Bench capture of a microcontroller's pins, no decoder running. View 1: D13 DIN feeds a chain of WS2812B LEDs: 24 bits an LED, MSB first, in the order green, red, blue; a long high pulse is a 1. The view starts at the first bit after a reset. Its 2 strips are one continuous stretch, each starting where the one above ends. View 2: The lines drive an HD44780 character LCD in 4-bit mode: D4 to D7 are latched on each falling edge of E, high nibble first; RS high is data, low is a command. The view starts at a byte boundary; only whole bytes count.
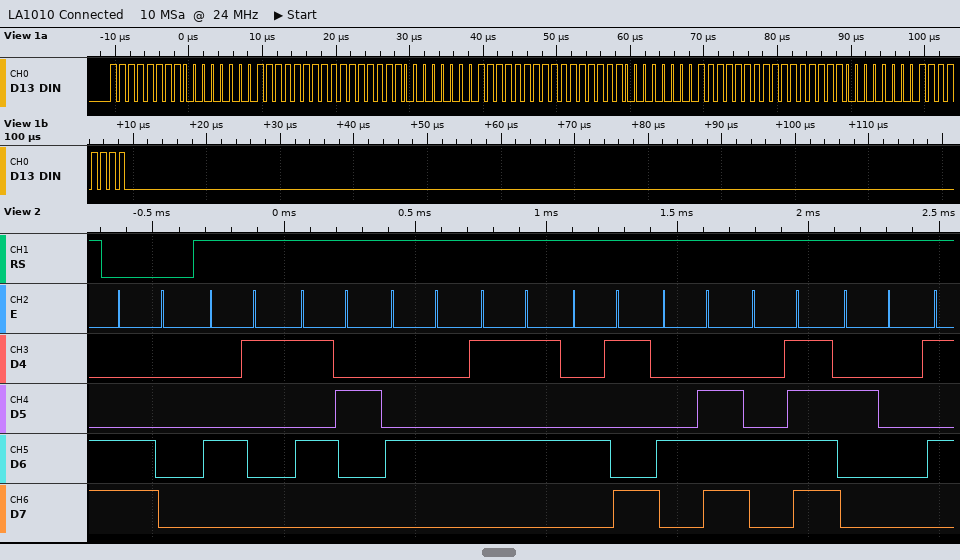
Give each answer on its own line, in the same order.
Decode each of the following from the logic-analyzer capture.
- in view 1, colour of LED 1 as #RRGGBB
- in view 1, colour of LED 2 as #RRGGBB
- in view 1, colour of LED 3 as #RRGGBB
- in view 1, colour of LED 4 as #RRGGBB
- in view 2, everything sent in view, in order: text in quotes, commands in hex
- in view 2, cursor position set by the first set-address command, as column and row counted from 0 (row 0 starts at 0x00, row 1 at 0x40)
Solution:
#00FFFF
#00FFFF
#00FFFF
#00FFFF
0xC0 "ARDUINO "
column 0, row 1
